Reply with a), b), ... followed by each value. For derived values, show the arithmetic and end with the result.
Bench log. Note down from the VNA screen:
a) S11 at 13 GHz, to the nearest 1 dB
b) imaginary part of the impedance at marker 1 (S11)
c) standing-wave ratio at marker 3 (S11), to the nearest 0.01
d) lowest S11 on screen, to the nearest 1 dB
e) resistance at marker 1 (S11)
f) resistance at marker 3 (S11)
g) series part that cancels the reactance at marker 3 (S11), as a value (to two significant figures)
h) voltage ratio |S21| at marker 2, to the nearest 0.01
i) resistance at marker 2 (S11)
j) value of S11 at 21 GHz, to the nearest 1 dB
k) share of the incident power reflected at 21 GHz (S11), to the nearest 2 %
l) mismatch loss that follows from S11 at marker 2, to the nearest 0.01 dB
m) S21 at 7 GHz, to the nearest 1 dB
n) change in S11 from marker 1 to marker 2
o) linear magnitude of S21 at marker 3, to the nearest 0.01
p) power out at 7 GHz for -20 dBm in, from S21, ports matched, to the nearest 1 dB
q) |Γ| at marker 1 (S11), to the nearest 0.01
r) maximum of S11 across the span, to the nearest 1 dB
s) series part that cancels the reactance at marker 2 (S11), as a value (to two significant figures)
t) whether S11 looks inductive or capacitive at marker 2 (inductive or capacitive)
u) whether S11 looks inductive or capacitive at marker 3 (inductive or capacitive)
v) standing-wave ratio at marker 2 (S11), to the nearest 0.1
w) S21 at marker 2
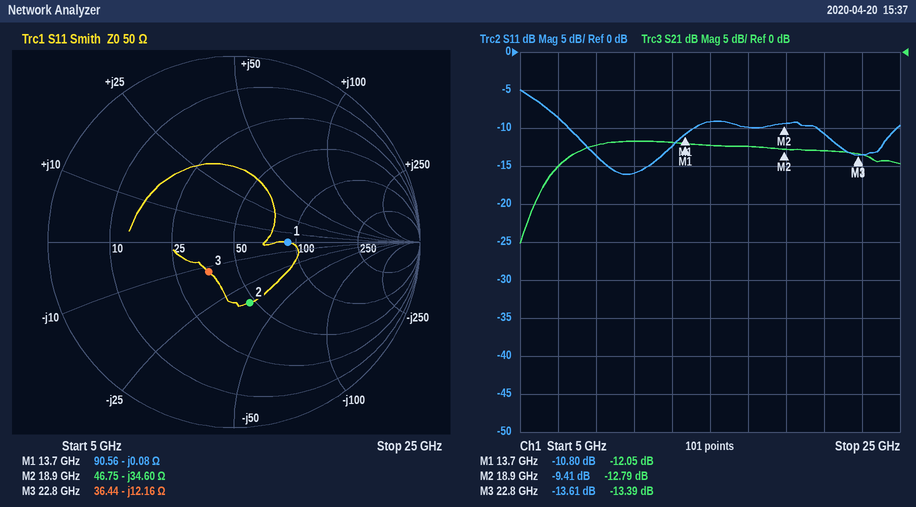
a) -12 dB
b) -0.08 Ω
c) 1.53
d) -16 dB
e) 90.56 Ω
f) 36.44 Ω
g) L = 12.16 Ω/(2π × 22.8 GHz) ≈ 85 pH
h) 10^(-12.79/20) ≈ 0.23
i) 46.75 Ω
j) -11 dB
k) 10^(-11/10) ≈ 8 %
l) −10 log10(1 − 10^(-9.41/10)) ≈ 0.53 dB
m) -15 dB
n) -9.41 − (-10.8) = 1.39 dB
o) 10^(-13.39/20) ≈ 0.21
p) -20 dBm + (-15 dB) = -35 dBm
q) 0.29
r) -5 dB
s) L = 34.6 Ω/(2π × 18.9 GHz) ≈ 291 pH, so 290 pH to two significant figures
t) capacitive
u) capacitive
v) 2.0
w) -12.79 dB
